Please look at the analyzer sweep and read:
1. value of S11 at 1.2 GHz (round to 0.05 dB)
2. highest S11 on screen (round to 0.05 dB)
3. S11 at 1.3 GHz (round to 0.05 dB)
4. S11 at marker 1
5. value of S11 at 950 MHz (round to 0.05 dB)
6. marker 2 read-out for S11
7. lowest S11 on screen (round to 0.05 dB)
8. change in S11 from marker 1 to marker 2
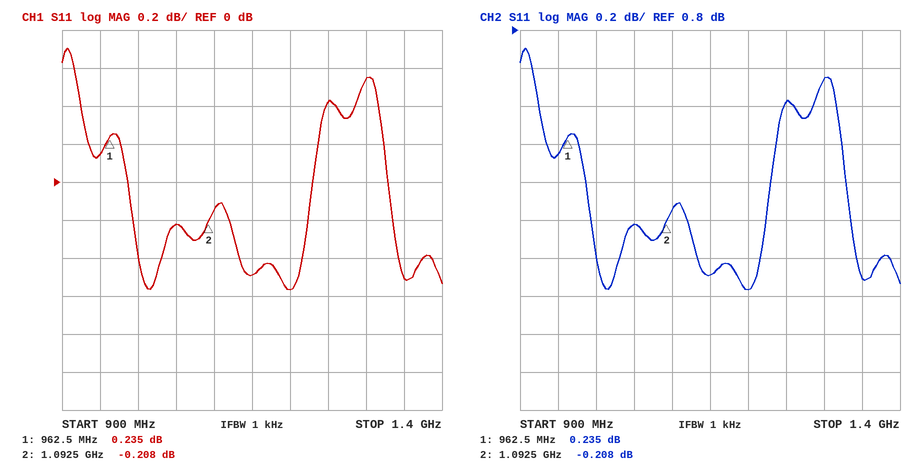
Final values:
-0.55 dB
0.70 dB
0.55 dB
0.235 dB
0.15 dB
-0.208 dB
-0.55 dB
-0.443 dB
